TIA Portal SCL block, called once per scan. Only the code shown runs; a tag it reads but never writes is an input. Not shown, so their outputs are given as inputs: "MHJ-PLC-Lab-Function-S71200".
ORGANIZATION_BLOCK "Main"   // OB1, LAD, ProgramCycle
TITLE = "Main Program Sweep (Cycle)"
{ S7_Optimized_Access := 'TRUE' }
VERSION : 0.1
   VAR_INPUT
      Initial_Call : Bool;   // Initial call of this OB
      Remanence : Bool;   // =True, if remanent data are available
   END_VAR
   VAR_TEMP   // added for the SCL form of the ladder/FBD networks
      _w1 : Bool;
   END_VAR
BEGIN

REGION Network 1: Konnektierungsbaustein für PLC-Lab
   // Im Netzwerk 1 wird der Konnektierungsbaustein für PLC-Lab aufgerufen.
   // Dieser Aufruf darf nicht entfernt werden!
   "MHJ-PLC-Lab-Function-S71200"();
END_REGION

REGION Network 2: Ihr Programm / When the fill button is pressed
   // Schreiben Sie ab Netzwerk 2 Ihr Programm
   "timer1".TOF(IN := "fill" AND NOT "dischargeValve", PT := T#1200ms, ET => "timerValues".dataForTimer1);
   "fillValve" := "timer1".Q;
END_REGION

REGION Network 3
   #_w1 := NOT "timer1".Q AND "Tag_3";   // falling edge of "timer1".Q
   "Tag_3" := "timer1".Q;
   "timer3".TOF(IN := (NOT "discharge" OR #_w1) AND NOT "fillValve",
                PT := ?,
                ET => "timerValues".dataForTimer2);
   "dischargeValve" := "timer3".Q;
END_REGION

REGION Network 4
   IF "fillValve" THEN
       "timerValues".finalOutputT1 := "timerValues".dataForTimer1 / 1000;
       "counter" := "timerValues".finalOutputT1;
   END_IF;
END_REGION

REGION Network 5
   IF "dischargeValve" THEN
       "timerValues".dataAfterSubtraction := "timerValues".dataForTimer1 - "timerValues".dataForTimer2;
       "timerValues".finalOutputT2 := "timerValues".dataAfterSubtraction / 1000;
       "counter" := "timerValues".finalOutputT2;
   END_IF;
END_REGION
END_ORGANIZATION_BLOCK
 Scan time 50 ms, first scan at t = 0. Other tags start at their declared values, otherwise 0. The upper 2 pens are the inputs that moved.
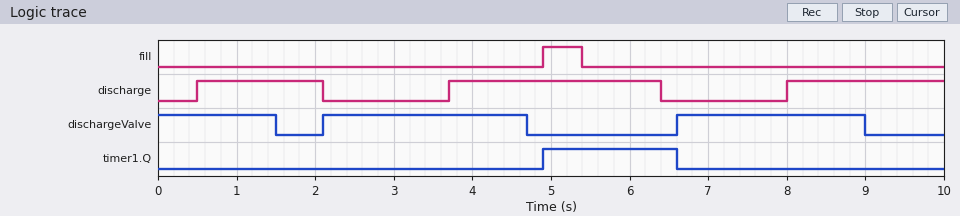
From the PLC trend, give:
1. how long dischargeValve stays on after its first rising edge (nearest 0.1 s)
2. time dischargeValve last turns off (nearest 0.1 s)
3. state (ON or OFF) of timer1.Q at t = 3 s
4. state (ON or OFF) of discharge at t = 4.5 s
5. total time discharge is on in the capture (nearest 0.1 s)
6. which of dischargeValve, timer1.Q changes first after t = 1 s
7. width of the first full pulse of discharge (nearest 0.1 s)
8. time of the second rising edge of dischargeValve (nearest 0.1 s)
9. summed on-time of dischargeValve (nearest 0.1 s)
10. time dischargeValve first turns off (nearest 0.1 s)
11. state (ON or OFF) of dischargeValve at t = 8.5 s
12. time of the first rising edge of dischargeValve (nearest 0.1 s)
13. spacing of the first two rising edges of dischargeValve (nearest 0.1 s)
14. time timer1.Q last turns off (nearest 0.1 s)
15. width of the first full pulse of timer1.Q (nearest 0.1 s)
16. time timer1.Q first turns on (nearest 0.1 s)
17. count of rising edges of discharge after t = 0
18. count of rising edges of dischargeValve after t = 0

2.6 s
9.0 s
OFF
ON
6.3 s
dischargeValve
1.6 s
6.6 s
6.5 s
1.5 s
ON
2.1 s
4.5 s
6.6 s
1.7 s
4.9 s
3
2
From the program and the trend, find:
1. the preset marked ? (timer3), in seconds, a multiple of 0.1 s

1.0 s
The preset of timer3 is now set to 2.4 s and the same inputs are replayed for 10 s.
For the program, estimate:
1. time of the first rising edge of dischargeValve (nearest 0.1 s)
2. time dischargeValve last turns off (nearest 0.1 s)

6.4 s
6.1 s
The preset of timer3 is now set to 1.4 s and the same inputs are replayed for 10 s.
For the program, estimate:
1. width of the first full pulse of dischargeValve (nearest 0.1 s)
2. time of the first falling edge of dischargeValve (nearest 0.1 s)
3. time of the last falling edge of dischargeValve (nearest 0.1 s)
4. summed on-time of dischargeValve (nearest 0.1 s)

3.0 s
1.9 s
9.4 s
7.7 s
